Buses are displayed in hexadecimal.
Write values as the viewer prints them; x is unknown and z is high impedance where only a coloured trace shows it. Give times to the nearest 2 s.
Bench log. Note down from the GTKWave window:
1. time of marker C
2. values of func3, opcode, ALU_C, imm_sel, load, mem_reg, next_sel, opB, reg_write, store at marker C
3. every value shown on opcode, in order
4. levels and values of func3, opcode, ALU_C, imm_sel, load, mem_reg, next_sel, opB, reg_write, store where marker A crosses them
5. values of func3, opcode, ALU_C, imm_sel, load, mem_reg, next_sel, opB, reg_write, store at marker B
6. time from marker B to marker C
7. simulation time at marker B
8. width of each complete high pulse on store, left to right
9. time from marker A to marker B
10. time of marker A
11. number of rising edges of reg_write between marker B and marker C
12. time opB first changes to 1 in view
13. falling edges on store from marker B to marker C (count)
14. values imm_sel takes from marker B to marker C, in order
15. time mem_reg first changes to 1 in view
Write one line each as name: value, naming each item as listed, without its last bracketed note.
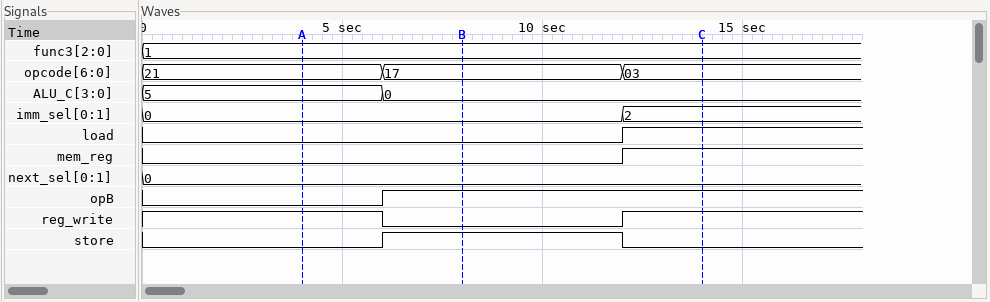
time of marker C: 14 s
values of func3, opcode, ALU_C, imm_sel, load, mem_reg, next_sel, opB, reg_write, store at marker C: func3=1, opcode=03, ALU_C=0, imm_sel=2, load=1, mem_reg=1, next_sel=0, opB=1, reg_write=1, store=0
every value shown on opcode, in order: 21, 17, 03
levels and values of func3, opcode, ALU_C, imm_sel, load, mem_reg, next_sel, opB, reg_write, store where marker A crosses them: func3=1, opcode=21, ALU_C=5, imm_sel=0, load=0, mem_reg=0, next_sel=0, opB=0, reg_write=1, store=0
values of func3, opcode, ALU_C, imm_sel, load, mem_reg, next_sel, opB, reg_write, store at marker B: func3=1, opcode=17, ALU_C=0, imm_sel=0, load=0, mem_reg=0, next_sel=0, opB=1, reg_write=0, store=1
time from marker B to marker C: 6 s
simulation time at marker B: 8 s
width of each complete high pulse on store, left to right: 6 s
time from marker A to marker B: 4 s
time of marker A: 4 s
number of rising edges of reg_write between marker B and marker C: 1
time opB first changes to 1 in view: 6 s
falling edges on store from marker B to marker C: 1
values imm_sel takes from marker B to marker C, in order: 0, 2
time mem_reg first changes to 1 in view: 12 s
